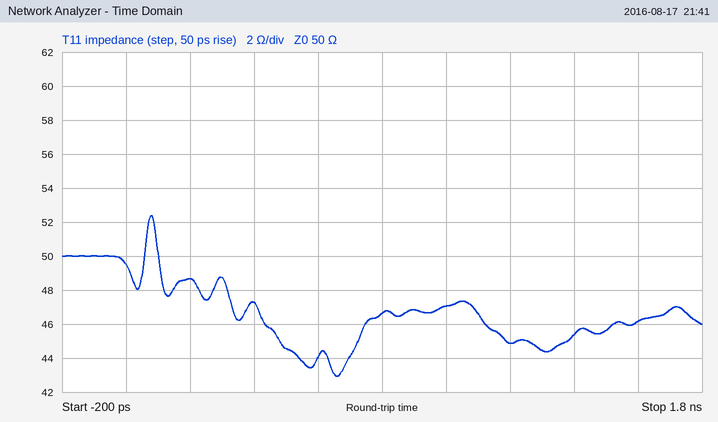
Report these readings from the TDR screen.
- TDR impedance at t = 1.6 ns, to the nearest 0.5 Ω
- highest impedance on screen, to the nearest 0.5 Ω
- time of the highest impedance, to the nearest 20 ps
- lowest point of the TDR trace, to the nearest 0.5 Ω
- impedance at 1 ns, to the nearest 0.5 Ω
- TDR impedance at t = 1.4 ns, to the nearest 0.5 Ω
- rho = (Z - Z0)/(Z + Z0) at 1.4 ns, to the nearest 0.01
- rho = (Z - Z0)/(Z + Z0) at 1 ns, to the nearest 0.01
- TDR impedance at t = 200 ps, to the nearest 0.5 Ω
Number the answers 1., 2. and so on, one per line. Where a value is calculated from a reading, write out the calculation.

1. 46.0 Ω
2. 52.5 Ω
3. 80 ps
4. 43.0 Ω
5. 47.0 Ω
6. 45.5 Ω
7. (45.5 − 50)/(45.5 + 50) ≈ -0.05
8. (47 − 50)/(47 + 50) ≈ -0.03
9. 48.5 Ω
